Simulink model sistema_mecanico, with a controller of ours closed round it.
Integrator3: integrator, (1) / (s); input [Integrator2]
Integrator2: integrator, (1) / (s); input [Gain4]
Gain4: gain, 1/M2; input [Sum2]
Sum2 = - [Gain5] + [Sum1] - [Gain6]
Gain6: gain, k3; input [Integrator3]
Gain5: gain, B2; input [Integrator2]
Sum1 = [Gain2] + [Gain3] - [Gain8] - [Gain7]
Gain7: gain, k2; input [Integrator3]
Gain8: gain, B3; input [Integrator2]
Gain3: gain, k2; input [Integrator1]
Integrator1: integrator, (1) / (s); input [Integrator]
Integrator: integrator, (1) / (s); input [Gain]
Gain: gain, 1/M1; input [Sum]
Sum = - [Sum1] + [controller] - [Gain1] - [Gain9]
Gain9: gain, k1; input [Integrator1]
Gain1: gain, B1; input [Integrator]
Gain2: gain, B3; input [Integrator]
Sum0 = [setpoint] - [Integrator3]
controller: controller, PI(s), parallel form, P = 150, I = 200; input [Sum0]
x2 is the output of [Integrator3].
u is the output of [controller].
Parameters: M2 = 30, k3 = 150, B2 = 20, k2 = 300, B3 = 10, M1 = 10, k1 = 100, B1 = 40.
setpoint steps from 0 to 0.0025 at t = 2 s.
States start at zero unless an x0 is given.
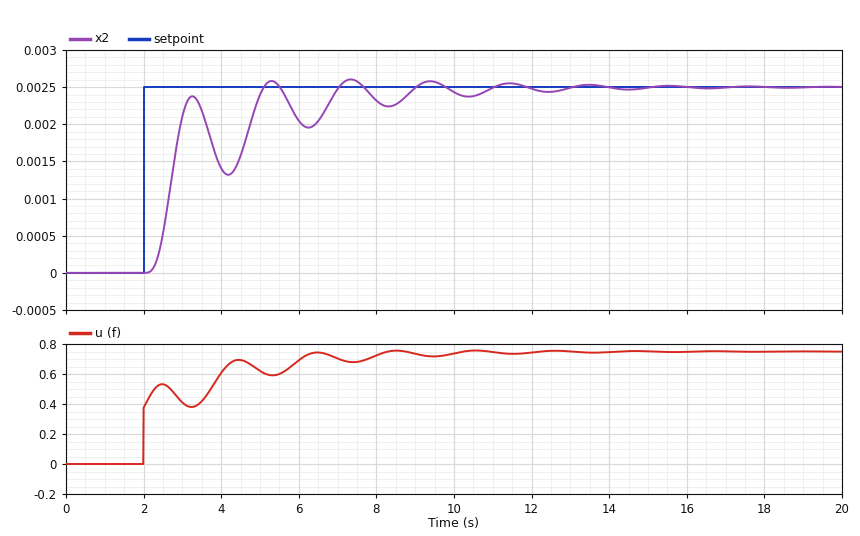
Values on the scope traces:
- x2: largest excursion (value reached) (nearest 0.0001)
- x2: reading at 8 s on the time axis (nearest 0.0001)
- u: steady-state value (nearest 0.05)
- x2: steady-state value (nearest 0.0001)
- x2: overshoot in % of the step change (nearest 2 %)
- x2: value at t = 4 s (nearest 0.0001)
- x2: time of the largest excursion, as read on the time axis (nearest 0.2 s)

0.0026
0.0023
0.75
0.0025
4 %
0.0014
7.4 s
